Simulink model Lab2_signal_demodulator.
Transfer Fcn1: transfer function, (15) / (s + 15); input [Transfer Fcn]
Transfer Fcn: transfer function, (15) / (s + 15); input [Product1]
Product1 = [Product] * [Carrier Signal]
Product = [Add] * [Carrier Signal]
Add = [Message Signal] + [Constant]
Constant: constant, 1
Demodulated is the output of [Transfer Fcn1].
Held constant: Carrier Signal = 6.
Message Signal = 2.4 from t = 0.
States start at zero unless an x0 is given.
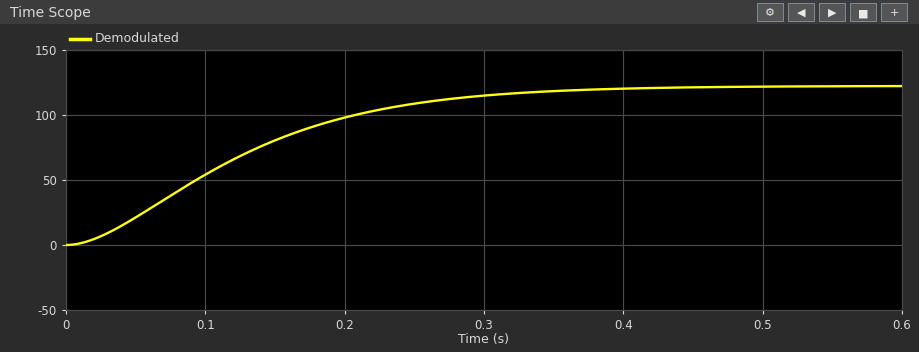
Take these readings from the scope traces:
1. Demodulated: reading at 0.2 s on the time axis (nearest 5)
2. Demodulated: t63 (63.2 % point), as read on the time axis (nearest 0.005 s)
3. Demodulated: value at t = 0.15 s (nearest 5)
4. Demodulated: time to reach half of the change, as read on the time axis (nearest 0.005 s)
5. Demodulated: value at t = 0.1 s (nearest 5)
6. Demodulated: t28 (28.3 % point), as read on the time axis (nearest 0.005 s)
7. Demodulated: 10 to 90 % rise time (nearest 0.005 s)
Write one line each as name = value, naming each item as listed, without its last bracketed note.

Demodulated: reading at 0.2 s on the time axis = 100
Demodulated: t63 (63.2 % point), as read on the time axis = 0.145 s
Demodulated: value at t = 0.15 s = 80
Demodulated: time to reach half of the change, as read on the time axis = 0.110 s
Demodulated: value at t = 0.1 s = 55
Demodulated: t28 (28.3 % point), as read on the time axis = 0.070 s
Demodulated: 10 to 90 % rise time = 0.225 s
